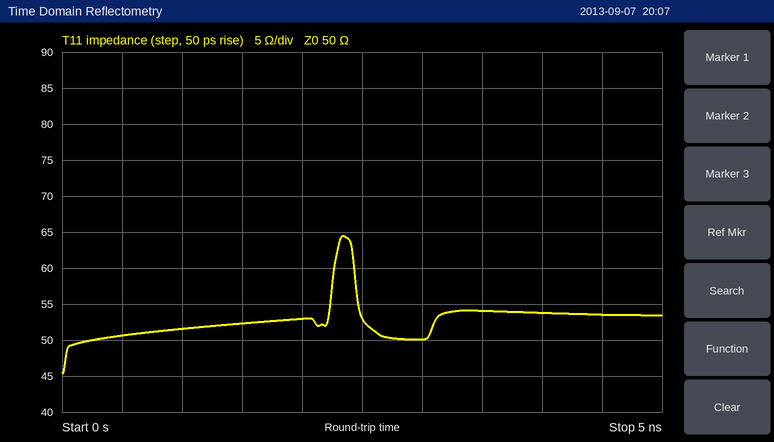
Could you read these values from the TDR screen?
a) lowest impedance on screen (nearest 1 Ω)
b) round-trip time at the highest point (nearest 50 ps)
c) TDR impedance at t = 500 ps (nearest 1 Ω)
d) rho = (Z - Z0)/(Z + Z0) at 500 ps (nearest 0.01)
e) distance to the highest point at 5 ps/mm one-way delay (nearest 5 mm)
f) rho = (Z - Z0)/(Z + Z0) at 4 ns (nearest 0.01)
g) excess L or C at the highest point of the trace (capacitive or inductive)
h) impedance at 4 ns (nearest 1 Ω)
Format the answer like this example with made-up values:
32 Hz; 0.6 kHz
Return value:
45 Ω; 2.35 ns; 51 Ω; +0.01; 235 mm; +0.04; inductive; 54 Ω
